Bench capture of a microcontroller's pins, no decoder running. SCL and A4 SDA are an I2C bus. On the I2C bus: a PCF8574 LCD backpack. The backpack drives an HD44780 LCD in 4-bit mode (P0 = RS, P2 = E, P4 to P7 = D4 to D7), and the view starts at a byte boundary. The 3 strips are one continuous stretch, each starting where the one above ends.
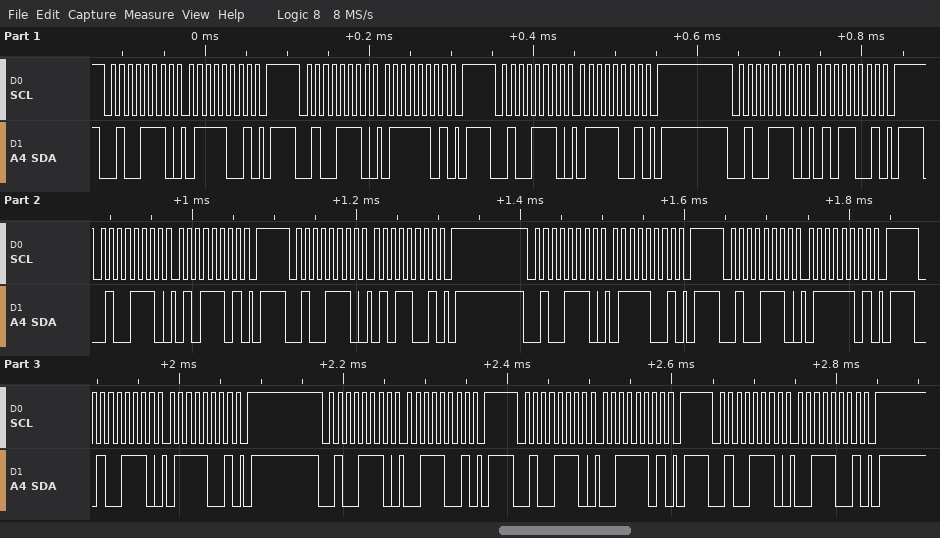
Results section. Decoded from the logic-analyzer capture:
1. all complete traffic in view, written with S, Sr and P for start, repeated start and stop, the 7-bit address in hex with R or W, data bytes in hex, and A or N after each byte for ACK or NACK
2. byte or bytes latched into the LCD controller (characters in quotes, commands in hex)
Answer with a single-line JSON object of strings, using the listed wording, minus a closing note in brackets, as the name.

{"all complete traffic in view, written with S, Sr and P for start, repeated start and stop, the 7-bit address in hex with R or W, data bytes in hex, and A or N after each byte for ACK or NACK": "S 27W A 79 A P S 27W A 7D A P S 27W A 79 A P S 27W A 59 A P S 27W A 5D A P S 27W A 59 A P S 27W A 79 A P S 27W A 7D A P S 27W A 79 A P S 27W A 39 A P S 27W A 3D A P S 27W A 39 A P", "byte or bytes latched into the LCD controller": "'u' 's'"}
